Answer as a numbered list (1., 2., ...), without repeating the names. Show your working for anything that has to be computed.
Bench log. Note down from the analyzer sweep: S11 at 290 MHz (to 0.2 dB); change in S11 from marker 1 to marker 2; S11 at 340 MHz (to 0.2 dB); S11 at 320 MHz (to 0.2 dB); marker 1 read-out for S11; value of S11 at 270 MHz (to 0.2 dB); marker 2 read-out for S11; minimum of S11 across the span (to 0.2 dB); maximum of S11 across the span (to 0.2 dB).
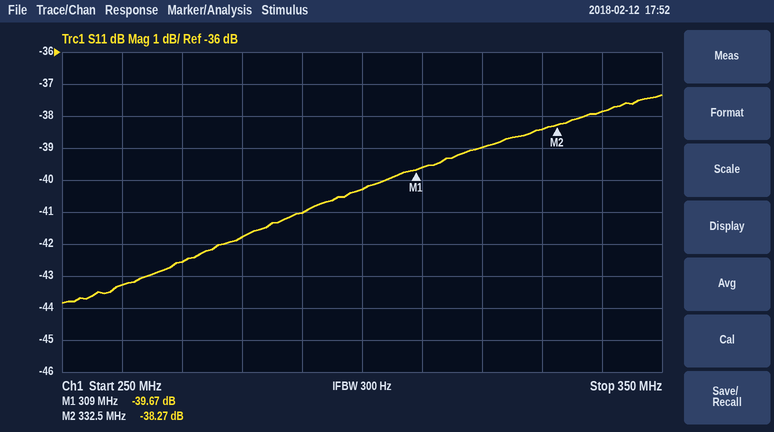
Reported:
1. -41.0 dB
2. -38.27 − (-39.67) = 1.40 dB
3. -37.8 dB
4. -39.0 dB
5. -39.67 dB
6. -42.6 dB
7. -38.27 dB
8. -43.8 dB
9. -37.4 dB
